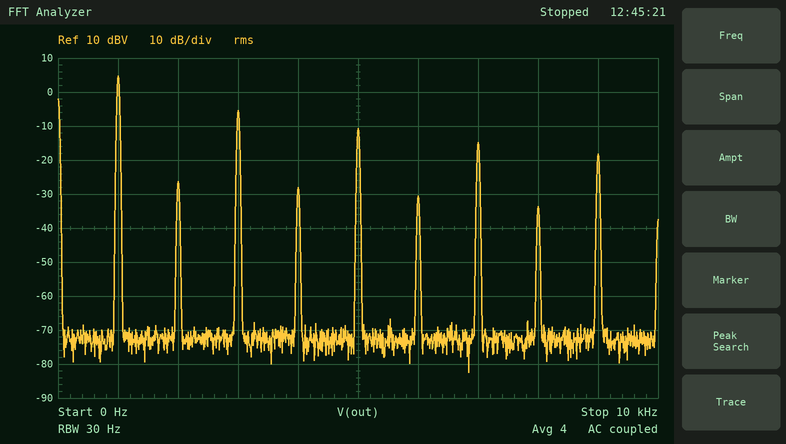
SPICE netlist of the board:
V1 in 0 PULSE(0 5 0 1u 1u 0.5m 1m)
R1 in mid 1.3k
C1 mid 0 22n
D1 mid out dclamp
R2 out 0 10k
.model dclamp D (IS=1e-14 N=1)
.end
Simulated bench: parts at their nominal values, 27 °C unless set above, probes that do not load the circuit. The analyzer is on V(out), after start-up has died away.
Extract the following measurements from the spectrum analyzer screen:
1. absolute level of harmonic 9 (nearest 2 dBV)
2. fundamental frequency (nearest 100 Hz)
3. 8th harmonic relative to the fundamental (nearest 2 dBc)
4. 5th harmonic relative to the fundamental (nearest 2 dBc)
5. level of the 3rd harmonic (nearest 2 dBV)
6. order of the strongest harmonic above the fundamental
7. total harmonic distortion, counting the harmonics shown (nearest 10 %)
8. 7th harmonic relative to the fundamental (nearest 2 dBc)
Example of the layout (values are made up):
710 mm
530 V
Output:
-18 dBV
1.0 kHz
-38 dBc
-16 dBc
-6 dBV
3
40 %
-20 dBc
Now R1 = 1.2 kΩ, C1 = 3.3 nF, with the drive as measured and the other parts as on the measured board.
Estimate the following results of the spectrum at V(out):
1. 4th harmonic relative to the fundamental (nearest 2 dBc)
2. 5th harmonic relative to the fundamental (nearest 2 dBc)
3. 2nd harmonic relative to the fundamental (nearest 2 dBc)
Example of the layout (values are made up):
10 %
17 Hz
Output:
-56 dBc
-14 dBc
-56 dBc
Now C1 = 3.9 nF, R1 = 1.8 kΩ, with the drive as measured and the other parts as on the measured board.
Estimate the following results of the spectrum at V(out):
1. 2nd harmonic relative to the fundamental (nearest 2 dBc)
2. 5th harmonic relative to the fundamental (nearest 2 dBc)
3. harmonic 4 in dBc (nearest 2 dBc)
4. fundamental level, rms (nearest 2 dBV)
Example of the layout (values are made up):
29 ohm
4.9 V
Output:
-46 dBc
-14 dBc
-46 dBc
4 dBV
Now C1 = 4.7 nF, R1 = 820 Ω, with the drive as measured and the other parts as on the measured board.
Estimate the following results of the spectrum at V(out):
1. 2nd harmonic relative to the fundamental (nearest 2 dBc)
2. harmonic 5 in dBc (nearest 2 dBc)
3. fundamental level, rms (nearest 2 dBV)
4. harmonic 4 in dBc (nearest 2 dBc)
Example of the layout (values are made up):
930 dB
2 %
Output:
-56 dBc
-14 dBc
6 dBV
-56 dBc
